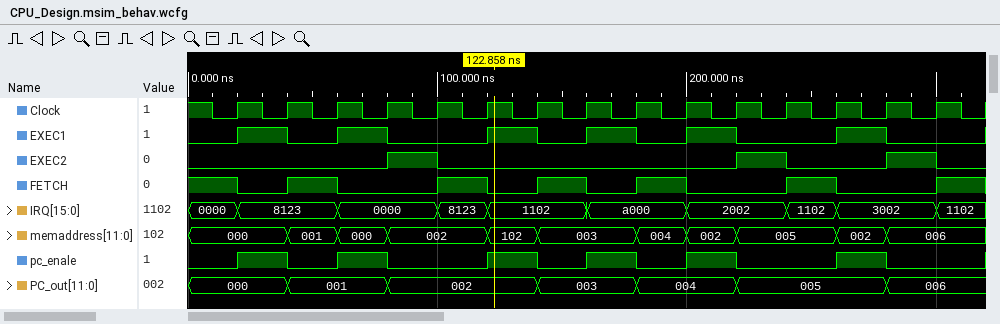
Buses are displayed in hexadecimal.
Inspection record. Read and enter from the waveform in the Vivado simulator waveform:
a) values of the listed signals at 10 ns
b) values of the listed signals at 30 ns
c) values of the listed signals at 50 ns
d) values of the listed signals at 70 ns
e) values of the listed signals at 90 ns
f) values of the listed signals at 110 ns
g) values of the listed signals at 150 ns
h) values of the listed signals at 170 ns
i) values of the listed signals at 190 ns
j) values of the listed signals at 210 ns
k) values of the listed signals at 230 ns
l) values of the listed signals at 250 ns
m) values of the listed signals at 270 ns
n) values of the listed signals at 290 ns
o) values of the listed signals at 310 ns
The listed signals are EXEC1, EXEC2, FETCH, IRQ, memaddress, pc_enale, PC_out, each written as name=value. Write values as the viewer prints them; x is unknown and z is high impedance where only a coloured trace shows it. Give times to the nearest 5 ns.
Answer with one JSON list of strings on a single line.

["EXEC1=0, EXEC2=0, FETCH=1, IRQ=0000, memaddress=000, pc_enale=0, PC_out=000", "EXEC1=1, EXEC2=0, FETCH=0, IRQ=8123, memaddress=000, pc_enale=1, PC_out=000", "EXEC1=0, EXEC2=0, FETCH=1, IRQ=8123, memaddress=001, pc_enale=0, PC_out=001", "EXEC1=1, EXEC2=0, FETCH=0, IRQ=0000, memaddress=000, pc_enale=1, PC_out=001", "EXEC1=0, EXEC2=1, FETCH=0, IRQ=0000, memaddress=002, pc_enale=0, PC_out=002", "EXEC1=0, EXEC2=0, FETCH=1, IRQ=8123, memaddress=002, pc_enale=0, PC_out=002", "EXEC1=0, EXEC2=0, FETCH=1, IRQ=1102, memaddress=003, pc_enale=0, PC_out=003", "EXEC1=1, EXEC2=0, FETCH=0, IRQ=a000, memaddress=003, pc_enale=1, PC_out=003", "EXEC1=0, EXEC2=0, FETCH=1, IRQ=a000, memaddress=004, pc_enale=0, PC_out=004", "EXEC1=1, EXEC2=0, FETCH=0, IRQ=2002, memaddress=002, pc_enale=1, PC_out=004", "EXEC1=0, EXEC2=1, FETCH=0, IRQ=2002, memaddress=005, pc_enale=0, PC_out=005", "EXEC1=0, EXEC2=0, FETCH=1, IRQ=1102, memaddress=005, pc_enale=0, PC_out=005", "EXEC1=1, EXEC2=0, FETCH=0, IRQ=3002, memaddress=002, pc_enale=1, PC_out=005", "EXEC1=0, EXEC2=1, FETCH=0, IRQ=3002, memaddress=006, pc_enale=0, PC_out=006", "EXEC1=0, EXEC2=0, FETCH=1, IRQ=1102, memaddress=006, pc_enale=0, PC_out=006"]
